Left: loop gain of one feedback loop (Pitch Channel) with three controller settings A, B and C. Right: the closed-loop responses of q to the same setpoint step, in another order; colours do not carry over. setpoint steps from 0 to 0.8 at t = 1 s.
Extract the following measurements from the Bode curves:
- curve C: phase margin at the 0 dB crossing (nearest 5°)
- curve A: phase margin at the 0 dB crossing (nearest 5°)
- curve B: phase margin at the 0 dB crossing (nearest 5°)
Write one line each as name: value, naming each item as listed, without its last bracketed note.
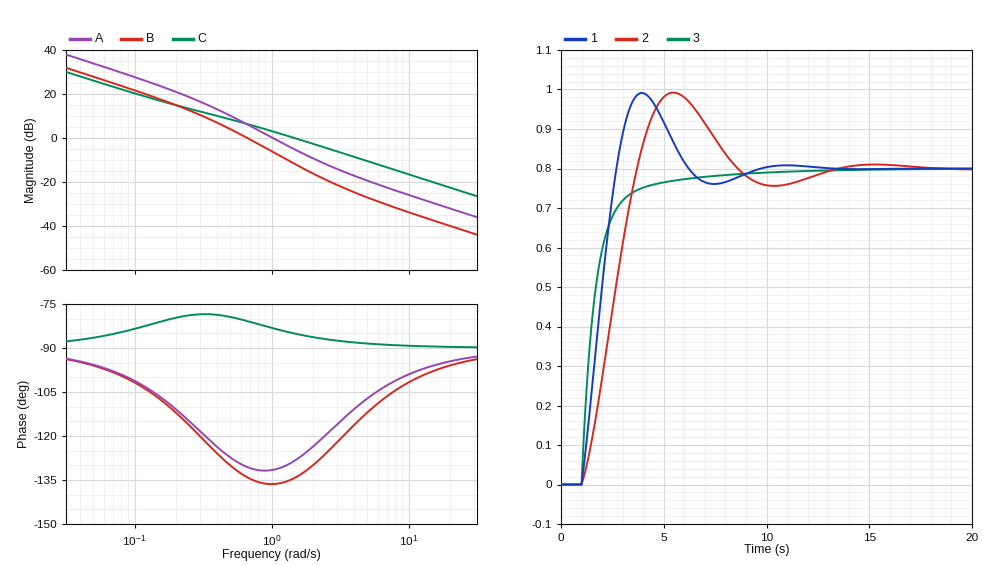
curve C: phase margin at the 0 dB crossing: 95°
curve A: phase margin at the 0 dB crossing: 50°
curve B: phase margin at the 0 dB crossing: 45°
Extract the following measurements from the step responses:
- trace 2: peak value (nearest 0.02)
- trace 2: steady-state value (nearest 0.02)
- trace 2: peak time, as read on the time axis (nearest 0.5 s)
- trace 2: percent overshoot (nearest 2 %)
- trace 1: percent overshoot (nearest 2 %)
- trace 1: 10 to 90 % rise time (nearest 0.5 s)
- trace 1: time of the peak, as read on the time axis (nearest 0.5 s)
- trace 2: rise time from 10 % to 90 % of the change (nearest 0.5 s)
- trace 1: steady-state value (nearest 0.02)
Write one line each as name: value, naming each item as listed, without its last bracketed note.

trace 2: peak value: 1.00
trace 2: steady-state value: 0.80
trace 2: peak time, as read on the time axis: 5.5 s
trace 2: percent overshoot: 24 %
trace 1: percent overshoot: 24 %
trace 1: 10 to 90 % rise time: 1.5 s
trace 1: time of the peak, as read on the time axis: 4.0 s
trace 2: rise time from 10 % to 90 % of the change: 2.0 s
trace 1: steady-state value: 0.80
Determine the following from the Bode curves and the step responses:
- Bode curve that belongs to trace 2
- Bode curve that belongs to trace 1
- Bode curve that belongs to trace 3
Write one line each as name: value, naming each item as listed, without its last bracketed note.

Bode curve that belongs to trace 2: B
Bode curve that belongs to trace 1: A
Bode curve that belongs to trace 3: C
